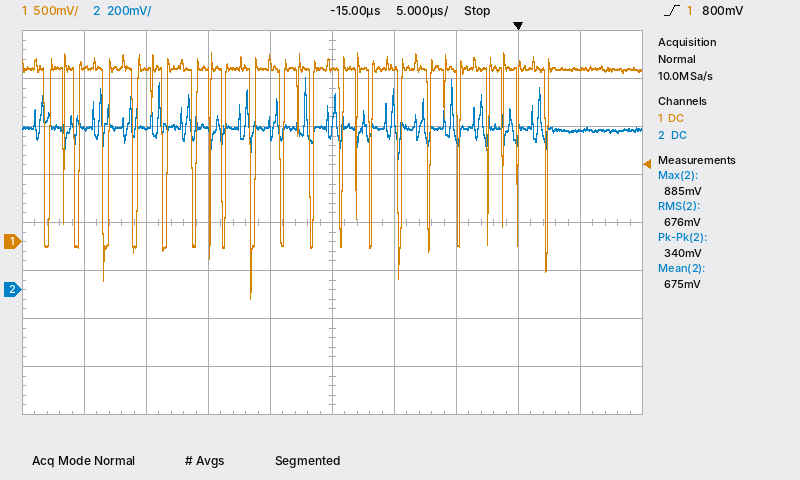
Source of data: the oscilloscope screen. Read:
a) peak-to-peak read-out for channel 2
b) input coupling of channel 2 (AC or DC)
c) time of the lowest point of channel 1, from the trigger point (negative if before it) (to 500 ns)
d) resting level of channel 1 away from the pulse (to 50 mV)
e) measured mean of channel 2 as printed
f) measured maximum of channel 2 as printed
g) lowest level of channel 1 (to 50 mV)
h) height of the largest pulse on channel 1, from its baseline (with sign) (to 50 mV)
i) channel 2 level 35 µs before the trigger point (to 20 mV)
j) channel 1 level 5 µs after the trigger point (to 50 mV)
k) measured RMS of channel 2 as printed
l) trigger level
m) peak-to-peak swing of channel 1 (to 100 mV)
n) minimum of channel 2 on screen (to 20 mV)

340 mV
DC
-21.5 µs
1.80 V
675 mV
885 mV
-600 mV
-2.40 V
680 mV
1.80 V
676 mV
800 mV
2.60 V
540 mV
